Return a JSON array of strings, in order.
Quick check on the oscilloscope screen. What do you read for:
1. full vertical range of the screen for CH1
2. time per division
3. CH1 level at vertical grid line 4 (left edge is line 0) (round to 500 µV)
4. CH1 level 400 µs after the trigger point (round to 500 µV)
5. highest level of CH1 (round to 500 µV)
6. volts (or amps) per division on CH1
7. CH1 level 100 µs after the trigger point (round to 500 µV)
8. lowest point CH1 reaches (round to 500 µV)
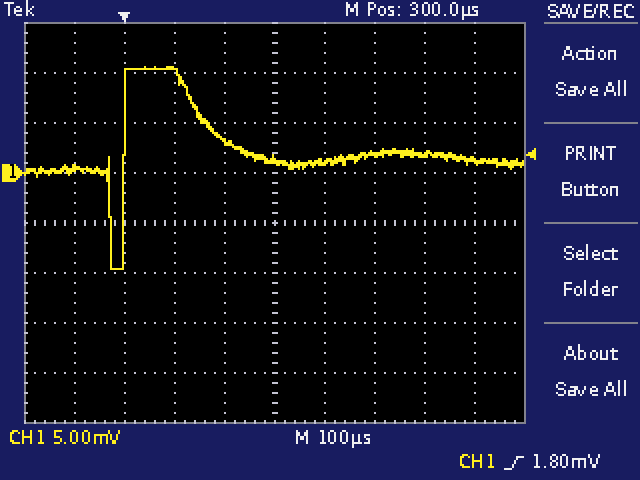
["40 mV", "100 µs", "3.0 mV", "1.0 mV", "10.5 mV", "5 mV", "10.0 mV", "-9.5 mV"]
